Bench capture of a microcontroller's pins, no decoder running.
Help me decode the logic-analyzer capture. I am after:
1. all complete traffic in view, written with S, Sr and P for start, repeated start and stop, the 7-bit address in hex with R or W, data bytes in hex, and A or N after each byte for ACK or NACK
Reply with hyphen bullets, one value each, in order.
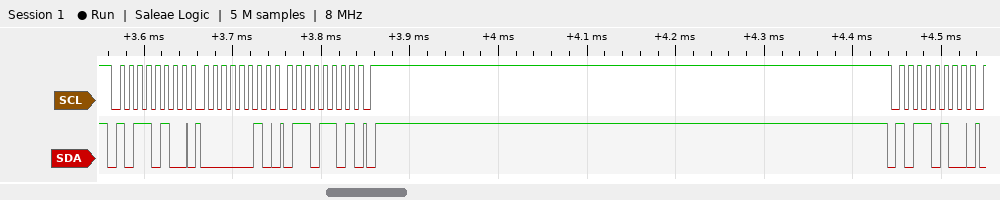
- S 5AW A 02 A 6D A P S 5AW A
